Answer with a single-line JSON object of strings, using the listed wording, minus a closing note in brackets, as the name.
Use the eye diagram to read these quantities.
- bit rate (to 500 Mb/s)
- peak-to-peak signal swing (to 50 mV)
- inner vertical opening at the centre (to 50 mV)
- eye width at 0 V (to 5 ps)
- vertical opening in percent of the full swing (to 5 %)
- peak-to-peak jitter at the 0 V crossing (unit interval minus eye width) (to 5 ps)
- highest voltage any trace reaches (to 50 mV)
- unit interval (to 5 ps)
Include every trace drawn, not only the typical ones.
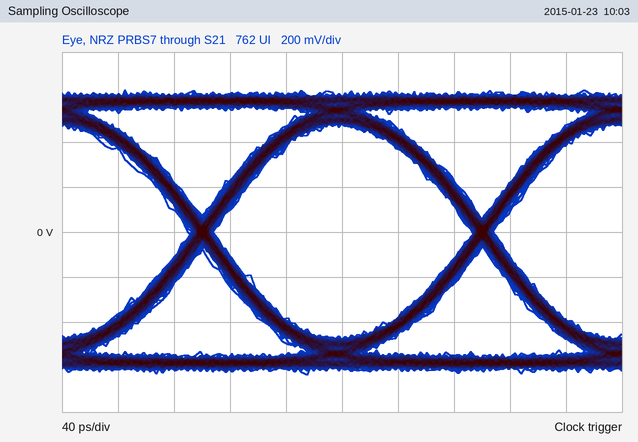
{"bit rate": "5.0 Gb/s", "peak-to-peak signal swing": "1.25 V", "inner vertical opening at the centre": "950 mV", "eye width at 0 V": "185 ps", "vertical opening in percent of the full swing": "75 %", "peak-to-peak jitter at the 0 V crossing (unit interval minus eye width)": "15 ps", "highest voltage any trace reaches": "650 mV", "unit interval": "200 ps"}
